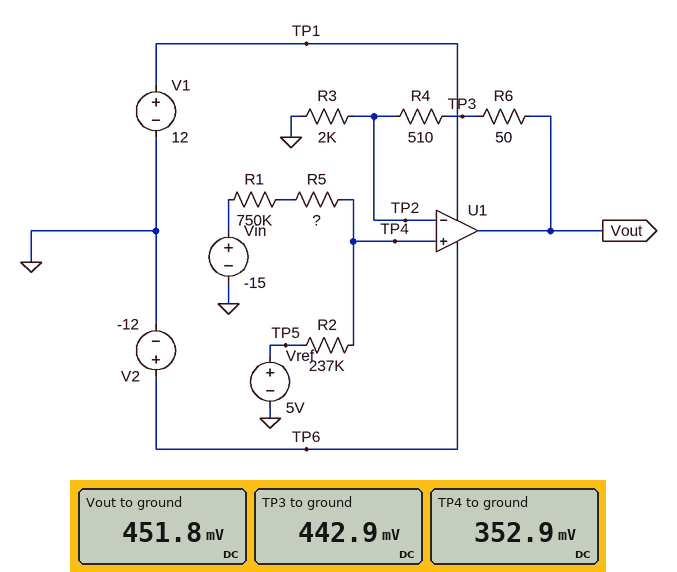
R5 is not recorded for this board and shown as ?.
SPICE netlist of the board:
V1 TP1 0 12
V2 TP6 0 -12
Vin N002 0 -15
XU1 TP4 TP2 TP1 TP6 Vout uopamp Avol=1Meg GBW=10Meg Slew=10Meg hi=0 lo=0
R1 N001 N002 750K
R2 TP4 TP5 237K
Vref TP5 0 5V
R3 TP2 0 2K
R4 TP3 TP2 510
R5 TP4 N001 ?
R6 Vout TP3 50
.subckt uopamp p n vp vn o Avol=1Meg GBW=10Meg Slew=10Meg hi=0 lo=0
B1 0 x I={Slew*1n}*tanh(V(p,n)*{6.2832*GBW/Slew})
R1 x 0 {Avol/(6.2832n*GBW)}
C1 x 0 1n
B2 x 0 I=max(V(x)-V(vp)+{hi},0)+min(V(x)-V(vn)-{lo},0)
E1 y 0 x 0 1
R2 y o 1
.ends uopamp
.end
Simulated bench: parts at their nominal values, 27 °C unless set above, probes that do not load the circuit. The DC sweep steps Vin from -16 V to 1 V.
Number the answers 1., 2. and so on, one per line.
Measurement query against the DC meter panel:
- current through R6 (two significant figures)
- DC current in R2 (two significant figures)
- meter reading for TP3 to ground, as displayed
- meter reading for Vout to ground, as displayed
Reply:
1. 180 µA
2. 20 µA
3. 442.9 mV
4. 451.8 mV
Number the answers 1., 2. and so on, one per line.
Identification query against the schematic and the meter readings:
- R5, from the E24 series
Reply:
1. 33 kΩ
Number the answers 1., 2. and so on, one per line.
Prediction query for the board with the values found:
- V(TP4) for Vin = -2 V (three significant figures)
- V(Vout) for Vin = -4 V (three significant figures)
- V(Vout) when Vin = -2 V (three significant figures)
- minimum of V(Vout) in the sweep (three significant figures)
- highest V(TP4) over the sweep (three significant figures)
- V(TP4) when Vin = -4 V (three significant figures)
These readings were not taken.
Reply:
1. 3.37 V
2. 3.72 V
3. 4.32 V
4. 154 mV
5. 4.07 V
6. 2.91 V
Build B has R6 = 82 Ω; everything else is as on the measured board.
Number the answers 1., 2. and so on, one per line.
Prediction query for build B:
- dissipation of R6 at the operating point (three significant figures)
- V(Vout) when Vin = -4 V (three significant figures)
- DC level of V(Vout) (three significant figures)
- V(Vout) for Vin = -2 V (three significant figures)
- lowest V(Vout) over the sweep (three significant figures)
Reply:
1. 2.55 µW
2. 3.77 V
3. 457 mV
4. 4.37 V
5. 156 mV
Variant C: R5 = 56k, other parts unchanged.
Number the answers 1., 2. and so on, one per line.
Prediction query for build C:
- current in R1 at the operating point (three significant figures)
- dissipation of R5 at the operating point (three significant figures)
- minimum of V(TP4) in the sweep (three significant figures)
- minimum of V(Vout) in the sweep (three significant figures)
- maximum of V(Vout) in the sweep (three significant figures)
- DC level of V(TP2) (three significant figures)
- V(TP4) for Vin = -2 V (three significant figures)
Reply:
1. 19.2 µA
2. 20.6 µW
3. 228 mV
4. 292 mV
5. 5.24 V
6. 455 mV
7. 3.41 V
